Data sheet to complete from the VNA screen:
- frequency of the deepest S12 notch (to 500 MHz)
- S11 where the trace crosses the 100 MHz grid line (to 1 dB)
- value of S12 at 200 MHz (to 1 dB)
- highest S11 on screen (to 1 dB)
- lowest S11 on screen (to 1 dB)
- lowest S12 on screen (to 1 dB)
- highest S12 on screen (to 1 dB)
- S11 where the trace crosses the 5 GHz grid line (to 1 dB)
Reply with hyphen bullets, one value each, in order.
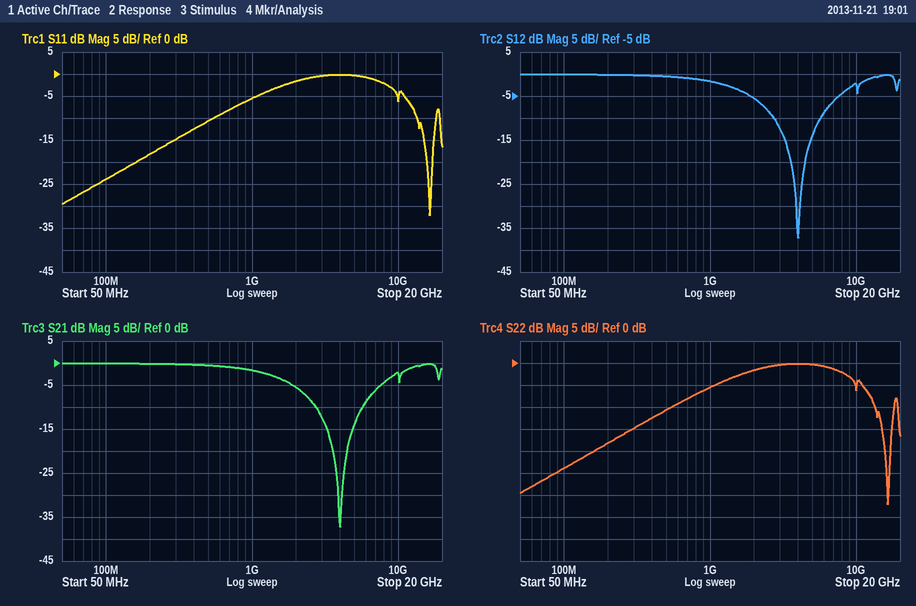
- 4.0 GHz
- -24 dB
- 0 dB
- 0 dB
- -32 dB
- -37 dB
- 0 dB
- 0 dB
